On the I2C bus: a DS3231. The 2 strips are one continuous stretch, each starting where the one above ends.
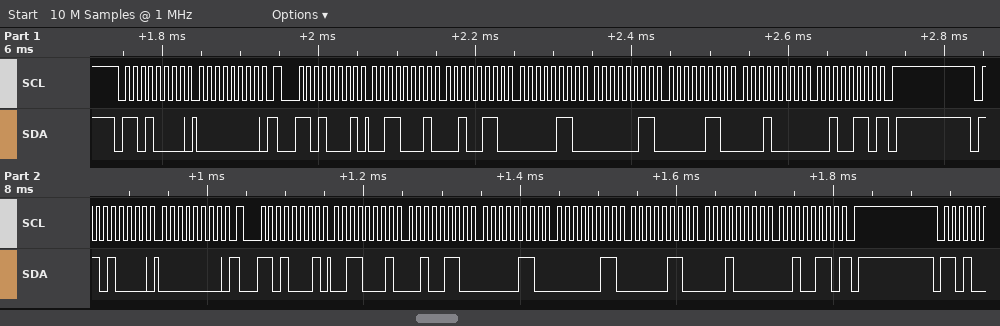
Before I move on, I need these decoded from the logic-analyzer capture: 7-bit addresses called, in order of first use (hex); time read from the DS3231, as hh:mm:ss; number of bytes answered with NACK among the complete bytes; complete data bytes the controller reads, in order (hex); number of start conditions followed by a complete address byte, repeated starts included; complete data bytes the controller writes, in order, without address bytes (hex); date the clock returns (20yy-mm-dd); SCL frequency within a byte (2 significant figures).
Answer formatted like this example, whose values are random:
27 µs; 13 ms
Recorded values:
0x68; 06:26:31; 2; 31 26 06 03 06 10 26 31 26 06 03 06 10 26; 4; 00 00; 2026-10-06; 100 kHz
